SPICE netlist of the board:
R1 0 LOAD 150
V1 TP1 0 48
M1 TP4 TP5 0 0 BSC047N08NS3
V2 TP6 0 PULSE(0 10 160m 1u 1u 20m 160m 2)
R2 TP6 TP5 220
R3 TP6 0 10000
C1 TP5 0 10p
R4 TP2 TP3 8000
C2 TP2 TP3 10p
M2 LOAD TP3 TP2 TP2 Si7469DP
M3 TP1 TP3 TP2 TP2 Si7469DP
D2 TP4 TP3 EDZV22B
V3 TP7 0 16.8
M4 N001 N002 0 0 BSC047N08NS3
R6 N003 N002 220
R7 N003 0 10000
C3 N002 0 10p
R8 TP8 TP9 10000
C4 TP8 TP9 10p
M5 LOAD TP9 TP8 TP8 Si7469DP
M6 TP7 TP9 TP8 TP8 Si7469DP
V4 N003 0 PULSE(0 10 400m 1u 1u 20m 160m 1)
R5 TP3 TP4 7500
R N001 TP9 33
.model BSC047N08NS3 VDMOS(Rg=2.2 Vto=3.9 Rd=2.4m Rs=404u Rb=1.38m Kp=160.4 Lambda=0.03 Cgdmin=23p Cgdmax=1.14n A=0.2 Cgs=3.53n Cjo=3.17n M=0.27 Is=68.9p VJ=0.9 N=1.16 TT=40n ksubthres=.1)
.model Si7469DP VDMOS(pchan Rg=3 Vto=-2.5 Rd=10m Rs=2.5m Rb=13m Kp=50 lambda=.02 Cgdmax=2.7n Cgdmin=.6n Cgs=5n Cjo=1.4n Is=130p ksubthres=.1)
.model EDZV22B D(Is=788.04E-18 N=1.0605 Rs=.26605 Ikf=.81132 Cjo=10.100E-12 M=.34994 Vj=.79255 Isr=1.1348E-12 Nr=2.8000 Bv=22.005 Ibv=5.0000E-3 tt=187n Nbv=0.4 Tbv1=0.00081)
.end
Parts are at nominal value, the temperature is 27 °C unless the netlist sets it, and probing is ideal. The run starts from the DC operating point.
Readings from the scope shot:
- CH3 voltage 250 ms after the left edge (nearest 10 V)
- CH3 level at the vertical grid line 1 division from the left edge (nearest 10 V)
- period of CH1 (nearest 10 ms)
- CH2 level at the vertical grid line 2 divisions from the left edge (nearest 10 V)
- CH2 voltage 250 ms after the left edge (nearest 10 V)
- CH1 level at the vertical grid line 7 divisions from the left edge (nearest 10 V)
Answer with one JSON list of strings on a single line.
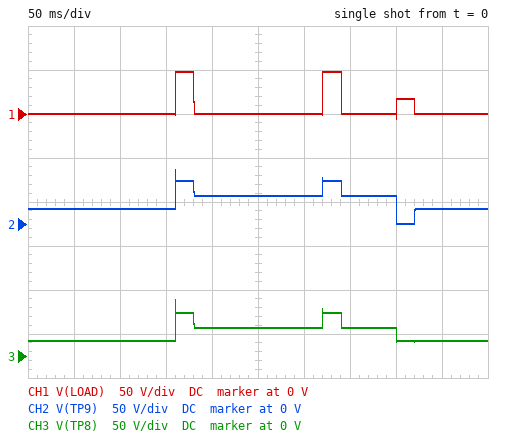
["30 V", "20 V", "160 ms", "20 V", "30 V", "0 V"]
